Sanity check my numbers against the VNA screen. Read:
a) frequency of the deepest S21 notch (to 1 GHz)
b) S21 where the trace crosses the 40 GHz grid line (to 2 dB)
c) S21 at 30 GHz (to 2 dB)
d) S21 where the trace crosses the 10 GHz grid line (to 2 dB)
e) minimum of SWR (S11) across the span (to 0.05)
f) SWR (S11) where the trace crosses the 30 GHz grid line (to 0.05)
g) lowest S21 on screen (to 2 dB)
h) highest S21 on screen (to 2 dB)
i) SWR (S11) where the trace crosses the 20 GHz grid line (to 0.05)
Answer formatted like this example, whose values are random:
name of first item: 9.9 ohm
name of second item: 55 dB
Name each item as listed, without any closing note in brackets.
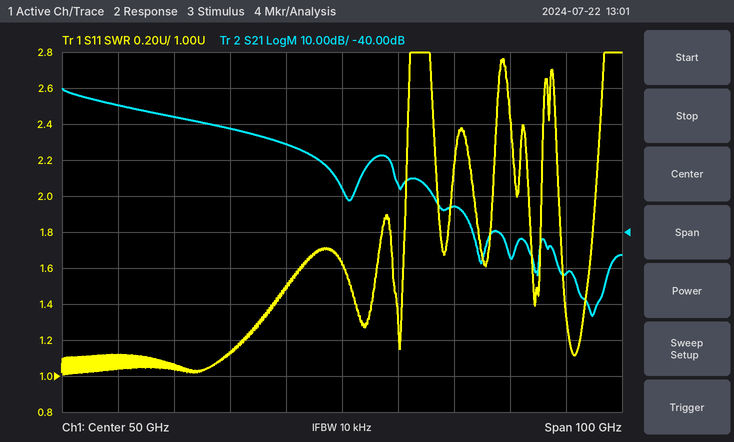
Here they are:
frequency of the deepest S21 notch: 95 GHz
S21 where the trace crosses the 40 GHz grid line: -16 dB
S21 at 30 GHz: -12 dB
S21 where the trace crosses the 10 GHz grid line: -4 dB
minimum of SWR (S11) across the span: 1.00
SWR (S11) where the trace crosses the 30 GHz grid line: 1.15
lowest S21 on screen: -64 dB
highest S21 on screen: 0 dB
SWR (S11) where the trace crosses the 20 GHz grid line: 1.05
